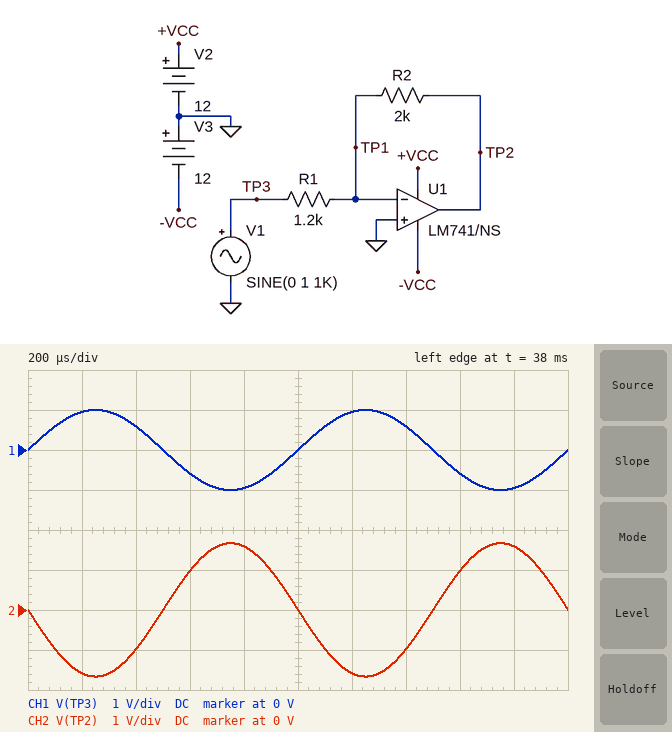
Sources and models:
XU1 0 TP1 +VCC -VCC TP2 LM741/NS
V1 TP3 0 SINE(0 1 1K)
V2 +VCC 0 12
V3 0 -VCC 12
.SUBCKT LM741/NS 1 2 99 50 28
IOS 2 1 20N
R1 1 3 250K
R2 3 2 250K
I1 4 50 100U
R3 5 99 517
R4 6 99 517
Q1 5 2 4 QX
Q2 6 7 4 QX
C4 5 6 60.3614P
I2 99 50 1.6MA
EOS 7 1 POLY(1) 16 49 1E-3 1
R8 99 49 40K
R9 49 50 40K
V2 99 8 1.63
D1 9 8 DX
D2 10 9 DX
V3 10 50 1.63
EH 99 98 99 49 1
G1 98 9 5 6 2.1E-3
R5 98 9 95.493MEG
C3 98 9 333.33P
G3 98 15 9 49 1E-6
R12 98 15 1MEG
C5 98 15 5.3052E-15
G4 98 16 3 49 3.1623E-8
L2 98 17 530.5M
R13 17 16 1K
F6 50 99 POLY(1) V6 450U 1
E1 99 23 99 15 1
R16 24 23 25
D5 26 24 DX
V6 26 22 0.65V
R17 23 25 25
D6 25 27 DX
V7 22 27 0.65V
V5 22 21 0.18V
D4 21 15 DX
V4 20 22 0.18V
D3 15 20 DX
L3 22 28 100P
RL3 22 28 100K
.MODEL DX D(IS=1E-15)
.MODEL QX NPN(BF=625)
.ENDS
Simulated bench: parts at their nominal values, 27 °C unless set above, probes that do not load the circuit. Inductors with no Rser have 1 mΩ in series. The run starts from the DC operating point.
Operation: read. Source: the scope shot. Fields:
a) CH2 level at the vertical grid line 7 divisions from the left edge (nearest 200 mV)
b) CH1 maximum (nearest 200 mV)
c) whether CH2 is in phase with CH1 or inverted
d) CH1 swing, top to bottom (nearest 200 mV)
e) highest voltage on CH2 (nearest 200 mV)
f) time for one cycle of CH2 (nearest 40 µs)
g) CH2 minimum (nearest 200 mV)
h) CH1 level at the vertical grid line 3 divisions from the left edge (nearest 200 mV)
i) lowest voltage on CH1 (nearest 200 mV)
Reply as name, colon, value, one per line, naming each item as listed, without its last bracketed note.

CH2 level at the vertical grid line 7 divisions from the left edge: -1.0 V
CH1 maximum: 1.0 V
whether CH2 is in phase with CH1 or inverted: inverted
CH1 swing, top to bottom: 2.0 V
highest voltage on CH2: 1.6 V
time for one cycle of CH2: 1.00 ms
CH2 minimum: -1.6 V
CH1 level at the vertical grid line 3 divisions from the left edge: -600 mV
lowest voltage on CH1: -1.0 V
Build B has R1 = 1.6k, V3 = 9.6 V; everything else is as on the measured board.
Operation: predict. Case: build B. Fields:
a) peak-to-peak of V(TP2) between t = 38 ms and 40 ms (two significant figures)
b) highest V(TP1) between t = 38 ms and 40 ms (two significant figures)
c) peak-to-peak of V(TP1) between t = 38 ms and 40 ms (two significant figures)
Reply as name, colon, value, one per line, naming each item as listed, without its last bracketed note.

peak-to-peak of V(TP2) between t = 38 ms and 40 ms: 2.5 V
highest V(TP1) between t = 38 ms and 40 ms: 2.3 mV
peak-to-peak of V(TP1) between t = 38 ms and 40 ms: 2.7 mV
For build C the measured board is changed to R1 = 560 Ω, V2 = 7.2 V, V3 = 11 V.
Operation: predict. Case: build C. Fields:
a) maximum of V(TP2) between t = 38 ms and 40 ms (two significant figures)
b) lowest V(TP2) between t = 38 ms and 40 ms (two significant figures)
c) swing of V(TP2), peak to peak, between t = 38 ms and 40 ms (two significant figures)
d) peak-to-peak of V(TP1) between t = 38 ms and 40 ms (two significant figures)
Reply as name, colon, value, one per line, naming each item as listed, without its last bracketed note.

maximum of V(TP2) between t = 38 ms and 40 ms: 3.6 V
lowest V(TP2) between t = 38 ms and 40 ms: -3.6 V
swing of V(TP2), peak to peak, between t = 38 ms and 40 ms: 7.1 V
peak-to-peak of V(TP1) between t = 38 ms and 40 ms: 7.8 mV
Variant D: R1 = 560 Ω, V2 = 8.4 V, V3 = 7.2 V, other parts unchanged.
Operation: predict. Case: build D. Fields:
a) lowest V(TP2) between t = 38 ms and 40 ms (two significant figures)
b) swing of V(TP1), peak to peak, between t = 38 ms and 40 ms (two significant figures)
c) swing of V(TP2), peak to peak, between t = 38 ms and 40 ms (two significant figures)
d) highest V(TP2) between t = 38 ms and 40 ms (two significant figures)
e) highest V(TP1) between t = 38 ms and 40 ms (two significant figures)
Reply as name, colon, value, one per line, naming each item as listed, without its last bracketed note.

lowest V(TP2) between t = 38 ms and 40 ms: -3.6 V
swing of V(TP1), peak to peak, between t = 38 ms and 40 ms: 7.8 mV
swing of V(TP2), peak to peak, between t = 38 ms and 40 ms: 7.1 V
highest V(TP2) between t = 38 ms and 40 ms: 3.6 V
highest V(TP1) between t = 38 ms and 40 ms: 4.9 mV
